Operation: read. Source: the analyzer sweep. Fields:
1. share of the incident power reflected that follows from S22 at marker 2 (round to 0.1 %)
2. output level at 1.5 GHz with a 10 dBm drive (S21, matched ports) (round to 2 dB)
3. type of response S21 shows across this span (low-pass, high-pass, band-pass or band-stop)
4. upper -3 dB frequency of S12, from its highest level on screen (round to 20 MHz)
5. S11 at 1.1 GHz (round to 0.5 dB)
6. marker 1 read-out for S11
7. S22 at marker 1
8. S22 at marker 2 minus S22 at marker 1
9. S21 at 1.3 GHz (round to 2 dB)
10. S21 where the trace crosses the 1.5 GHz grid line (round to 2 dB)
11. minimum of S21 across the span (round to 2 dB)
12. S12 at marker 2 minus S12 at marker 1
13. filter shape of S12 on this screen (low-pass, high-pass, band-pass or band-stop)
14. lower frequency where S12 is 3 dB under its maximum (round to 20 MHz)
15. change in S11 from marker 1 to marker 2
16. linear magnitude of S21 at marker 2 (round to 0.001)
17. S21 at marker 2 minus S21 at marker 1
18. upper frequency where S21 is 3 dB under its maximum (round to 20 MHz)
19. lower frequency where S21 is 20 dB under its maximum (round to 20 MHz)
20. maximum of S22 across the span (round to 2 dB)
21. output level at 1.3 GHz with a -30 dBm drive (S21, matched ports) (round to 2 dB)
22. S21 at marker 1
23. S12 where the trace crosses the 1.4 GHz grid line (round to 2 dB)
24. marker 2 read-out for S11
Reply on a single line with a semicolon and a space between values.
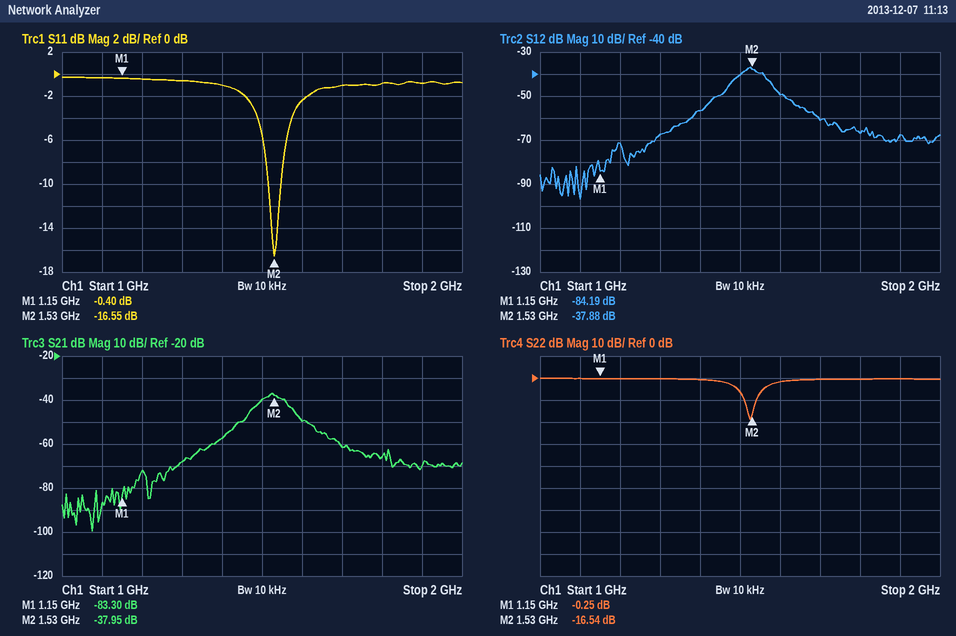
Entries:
2.2 %; -30 dBm; band-pass; 1.56 GHz; -0.5 dB; -0.40 dB; -0.25 dB; -16.29 dB; -68 dB; -40 dB; -100 dB; 46.31 dB; band-pass; 1.50 GHz; -16.15 dB; 0.013; 45.35 dB; 1.56 GHz; 1.40 GHz; 0 dB; -98 dBm; -83.30 dB; -56 dB; -16.55 dB
